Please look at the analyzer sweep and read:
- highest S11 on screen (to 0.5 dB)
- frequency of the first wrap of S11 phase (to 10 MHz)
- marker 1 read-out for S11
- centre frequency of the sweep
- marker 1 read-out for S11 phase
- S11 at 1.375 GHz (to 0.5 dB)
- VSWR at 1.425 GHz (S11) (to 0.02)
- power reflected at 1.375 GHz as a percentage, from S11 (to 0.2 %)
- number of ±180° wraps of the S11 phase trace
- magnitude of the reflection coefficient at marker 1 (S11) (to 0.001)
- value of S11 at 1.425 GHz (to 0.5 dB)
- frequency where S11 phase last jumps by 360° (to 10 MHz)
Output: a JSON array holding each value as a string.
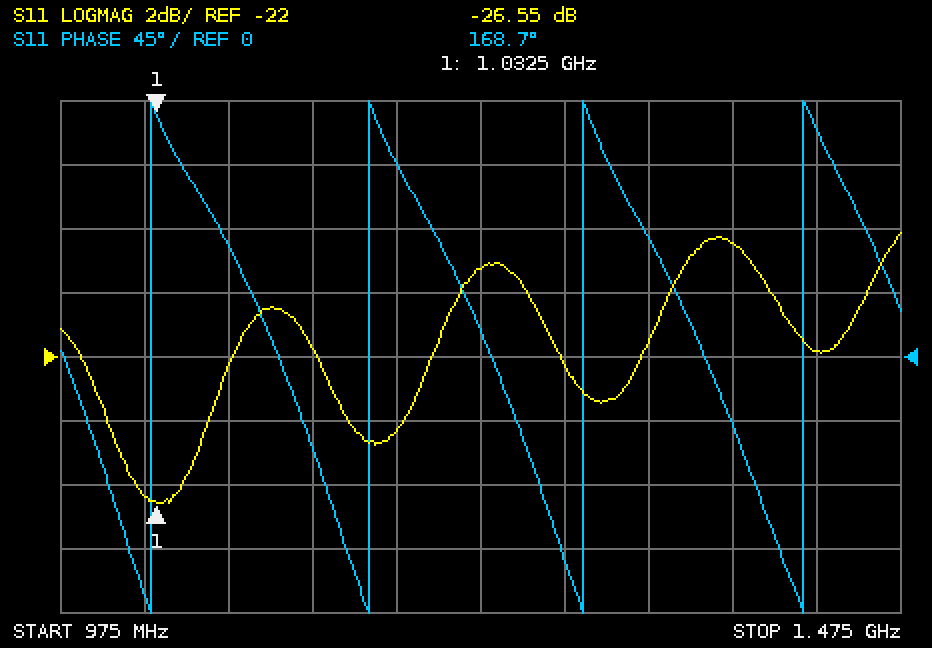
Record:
["-18.0 dB", "1.03 GHz", "-26.55 dB", "1.225 GHz", "168.7°", "-18.5 dB", "1.18", "1.4 %", "4", "0.047", "-22.0 dB", "1.42 GHz"]
